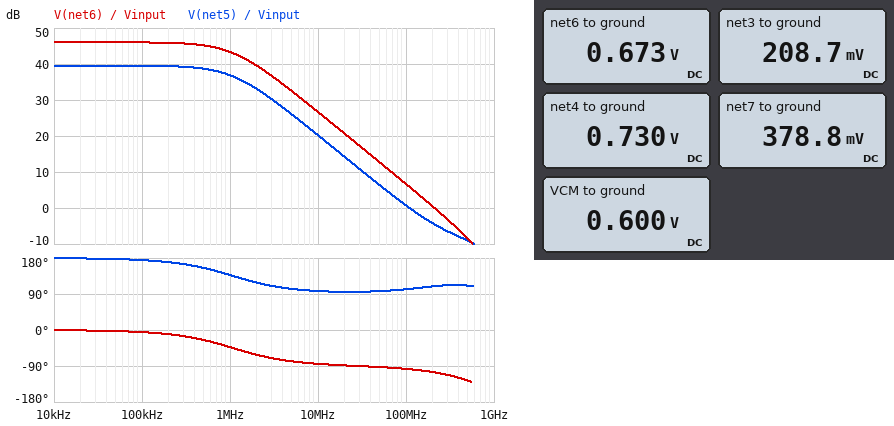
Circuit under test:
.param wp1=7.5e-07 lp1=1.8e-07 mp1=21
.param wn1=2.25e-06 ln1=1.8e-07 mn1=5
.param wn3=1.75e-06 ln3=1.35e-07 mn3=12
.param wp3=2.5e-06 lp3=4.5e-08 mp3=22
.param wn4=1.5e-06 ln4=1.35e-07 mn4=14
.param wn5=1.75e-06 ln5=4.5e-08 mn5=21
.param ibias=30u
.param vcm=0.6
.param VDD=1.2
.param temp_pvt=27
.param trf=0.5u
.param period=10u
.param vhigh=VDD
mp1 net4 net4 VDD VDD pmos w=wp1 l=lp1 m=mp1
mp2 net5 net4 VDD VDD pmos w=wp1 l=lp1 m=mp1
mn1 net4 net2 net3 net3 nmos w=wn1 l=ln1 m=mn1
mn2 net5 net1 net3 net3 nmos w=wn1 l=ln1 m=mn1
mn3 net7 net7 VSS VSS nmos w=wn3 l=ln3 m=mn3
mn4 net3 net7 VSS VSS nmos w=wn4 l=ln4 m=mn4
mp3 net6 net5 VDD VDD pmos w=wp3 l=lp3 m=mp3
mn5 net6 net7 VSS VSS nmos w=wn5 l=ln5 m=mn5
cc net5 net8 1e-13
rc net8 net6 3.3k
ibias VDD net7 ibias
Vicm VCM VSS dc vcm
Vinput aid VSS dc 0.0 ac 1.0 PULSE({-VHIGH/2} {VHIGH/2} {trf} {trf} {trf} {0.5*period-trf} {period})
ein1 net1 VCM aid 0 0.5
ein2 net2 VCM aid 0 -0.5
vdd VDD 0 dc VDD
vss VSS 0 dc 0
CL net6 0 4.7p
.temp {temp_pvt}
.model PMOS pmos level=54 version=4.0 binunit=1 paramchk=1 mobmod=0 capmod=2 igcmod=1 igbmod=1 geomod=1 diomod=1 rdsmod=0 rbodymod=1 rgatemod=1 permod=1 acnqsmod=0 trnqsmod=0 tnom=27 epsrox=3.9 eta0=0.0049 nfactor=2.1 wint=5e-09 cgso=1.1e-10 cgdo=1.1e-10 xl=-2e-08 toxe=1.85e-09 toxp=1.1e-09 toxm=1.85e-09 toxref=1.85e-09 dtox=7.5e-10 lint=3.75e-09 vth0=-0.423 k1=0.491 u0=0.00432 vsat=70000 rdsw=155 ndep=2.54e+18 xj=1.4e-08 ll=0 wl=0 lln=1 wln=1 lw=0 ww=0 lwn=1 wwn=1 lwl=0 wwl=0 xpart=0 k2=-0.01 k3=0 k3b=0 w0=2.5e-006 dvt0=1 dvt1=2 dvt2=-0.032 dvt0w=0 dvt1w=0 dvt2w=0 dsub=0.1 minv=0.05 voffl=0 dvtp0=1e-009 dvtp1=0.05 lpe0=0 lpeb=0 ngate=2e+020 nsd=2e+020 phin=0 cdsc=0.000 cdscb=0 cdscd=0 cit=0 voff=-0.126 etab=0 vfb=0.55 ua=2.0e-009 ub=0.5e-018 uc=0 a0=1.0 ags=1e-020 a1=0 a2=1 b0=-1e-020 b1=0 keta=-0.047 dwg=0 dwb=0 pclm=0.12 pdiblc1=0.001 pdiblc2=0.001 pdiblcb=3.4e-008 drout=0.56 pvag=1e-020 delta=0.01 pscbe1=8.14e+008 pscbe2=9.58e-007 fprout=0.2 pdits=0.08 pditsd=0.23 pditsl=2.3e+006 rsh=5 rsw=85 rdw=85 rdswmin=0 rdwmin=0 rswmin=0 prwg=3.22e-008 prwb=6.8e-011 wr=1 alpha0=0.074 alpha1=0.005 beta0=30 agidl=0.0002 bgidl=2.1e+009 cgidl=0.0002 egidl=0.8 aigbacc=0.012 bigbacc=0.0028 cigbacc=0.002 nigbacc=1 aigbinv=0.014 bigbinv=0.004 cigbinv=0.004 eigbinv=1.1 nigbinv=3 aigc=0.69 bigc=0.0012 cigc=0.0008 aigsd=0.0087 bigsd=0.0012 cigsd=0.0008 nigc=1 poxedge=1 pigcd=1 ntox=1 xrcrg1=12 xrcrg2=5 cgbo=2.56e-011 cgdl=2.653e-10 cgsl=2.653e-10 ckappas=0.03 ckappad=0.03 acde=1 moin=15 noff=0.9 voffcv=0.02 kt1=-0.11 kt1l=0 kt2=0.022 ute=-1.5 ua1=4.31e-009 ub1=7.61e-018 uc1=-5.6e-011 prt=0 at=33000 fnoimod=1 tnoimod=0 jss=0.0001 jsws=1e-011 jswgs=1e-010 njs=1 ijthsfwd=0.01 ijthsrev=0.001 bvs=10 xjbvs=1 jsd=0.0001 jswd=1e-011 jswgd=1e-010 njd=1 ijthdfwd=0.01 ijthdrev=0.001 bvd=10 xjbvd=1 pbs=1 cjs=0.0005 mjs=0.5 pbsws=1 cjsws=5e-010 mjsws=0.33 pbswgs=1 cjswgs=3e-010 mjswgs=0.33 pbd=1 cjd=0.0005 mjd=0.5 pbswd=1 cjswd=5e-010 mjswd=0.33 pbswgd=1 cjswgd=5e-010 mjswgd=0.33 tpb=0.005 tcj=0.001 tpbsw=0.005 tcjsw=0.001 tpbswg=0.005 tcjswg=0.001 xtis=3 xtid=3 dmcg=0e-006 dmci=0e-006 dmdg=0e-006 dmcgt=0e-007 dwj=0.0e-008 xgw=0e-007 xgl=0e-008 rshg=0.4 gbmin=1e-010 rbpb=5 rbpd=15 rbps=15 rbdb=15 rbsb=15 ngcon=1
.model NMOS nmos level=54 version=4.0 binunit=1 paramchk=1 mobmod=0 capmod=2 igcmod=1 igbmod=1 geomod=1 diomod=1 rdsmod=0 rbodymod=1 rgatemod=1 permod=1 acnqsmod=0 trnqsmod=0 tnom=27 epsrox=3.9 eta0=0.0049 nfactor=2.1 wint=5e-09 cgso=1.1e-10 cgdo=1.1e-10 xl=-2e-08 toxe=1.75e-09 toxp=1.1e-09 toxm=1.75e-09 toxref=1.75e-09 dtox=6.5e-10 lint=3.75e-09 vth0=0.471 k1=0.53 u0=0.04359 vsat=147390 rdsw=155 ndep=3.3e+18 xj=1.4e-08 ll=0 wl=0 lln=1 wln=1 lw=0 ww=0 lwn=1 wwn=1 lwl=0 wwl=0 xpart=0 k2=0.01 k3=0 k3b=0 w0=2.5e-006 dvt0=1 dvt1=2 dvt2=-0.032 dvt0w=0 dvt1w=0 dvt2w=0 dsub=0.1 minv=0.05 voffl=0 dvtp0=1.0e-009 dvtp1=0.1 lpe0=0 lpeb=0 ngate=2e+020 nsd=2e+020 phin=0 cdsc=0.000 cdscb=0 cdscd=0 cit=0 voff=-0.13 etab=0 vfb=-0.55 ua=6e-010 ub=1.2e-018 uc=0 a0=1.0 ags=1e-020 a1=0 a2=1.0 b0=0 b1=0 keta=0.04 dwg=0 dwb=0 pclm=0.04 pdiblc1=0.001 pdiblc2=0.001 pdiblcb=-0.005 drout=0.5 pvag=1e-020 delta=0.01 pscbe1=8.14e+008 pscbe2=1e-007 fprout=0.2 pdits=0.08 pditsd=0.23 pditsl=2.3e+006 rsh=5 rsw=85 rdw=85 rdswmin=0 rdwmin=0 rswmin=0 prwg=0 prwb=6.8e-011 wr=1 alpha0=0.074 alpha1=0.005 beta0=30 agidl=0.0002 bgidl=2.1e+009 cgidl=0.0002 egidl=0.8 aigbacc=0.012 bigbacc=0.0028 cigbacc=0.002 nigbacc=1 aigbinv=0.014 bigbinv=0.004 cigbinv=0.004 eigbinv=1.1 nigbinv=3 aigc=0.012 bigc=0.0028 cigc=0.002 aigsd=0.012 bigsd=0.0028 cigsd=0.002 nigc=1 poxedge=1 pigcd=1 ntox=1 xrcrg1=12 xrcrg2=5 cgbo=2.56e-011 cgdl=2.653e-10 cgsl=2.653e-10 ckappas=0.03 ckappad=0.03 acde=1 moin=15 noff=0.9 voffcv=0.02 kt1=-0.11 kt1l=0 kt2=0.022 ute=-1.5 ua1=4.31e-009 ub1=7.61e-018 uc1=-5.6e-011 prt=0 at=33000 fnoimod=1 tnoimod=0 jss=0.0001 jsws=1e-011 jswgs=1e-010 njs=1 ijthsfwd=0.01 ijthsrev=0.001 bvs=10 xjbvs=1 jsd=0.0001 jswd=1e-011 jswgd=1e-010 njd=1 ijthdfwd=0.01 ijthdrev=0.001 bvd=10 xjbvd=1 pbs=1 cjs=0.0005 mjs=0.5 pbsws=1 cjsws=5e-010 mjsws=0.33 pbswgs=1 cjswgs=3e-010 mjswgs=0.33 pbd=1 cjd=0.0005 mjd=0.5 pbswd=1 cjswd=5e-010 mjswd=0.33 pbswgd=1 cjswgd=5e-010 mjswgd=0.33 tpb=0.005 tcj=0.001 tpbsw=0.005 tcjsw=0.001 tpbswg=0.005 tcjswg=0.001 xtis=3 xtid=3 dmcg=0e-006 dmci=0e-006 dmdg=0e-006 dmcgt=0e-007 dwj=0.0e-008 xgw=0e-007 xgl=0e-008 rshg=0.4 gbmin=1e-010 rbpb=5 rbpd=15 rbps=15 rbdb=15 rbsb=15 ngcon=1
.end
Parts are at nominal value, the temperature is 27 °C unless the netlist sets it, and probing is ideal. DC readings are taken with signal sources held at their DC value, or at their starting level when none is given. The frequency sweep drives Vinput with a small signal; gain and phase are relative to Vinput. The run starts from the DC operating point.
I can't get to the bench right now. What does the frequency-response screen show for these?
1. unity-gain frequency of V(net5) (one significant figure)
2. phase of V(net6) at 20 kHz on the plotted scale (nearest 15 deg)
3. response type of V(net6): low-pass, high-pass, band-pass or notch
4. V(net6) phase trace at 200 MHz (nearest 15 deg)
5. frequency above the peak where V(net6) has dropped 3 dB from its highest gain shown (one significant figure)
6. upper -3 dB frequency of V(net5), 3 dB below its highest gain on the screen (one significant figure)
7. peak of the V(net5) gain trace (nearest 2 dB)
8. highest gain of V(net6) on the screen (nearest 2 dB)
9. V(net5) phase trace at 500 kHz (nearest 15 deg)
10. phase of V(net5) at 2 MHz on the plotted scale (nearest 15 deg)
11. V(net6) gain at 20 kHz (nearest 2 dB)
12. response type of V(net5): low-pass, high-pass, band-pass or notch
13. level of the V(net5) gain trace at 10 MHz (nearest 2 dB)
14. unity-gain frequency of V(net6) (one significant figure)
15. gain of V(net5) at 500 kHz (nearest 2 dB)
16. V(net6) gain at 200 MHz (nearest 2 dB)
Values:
100 MHz
0 deg
low-pass
-105 deg
1 MHz
1 MHz
40 dB
46 dB
150 deg
120 deg
46 dB
low-pass
20 dB
200 MHz
38 dB
0 dB
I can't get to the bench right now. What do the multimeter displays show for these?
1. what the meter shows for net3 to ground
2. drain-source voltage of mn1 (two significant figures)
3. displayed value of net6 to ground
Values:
208.7 mV
520 mV
0.673 V
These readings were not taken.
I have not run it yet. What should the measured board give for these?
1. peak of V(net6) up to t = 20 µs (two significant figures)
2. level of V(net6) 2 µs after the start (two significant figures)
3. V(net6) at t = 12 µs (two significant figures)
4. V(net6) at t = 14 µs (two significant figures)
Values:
1.1 V
1.1 V
1.1 V
1.1 V
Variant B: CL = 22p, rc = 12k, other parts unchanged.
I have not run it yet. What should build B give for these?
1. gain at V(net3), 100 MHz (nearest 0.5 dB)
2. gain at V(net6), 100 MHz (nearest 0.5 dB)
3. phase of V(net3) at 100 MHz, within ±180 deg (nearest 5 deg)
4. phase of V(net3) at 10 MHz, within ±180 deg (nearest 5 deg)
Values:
-29.5 dB
7.0 dB
160 deg
145 deg
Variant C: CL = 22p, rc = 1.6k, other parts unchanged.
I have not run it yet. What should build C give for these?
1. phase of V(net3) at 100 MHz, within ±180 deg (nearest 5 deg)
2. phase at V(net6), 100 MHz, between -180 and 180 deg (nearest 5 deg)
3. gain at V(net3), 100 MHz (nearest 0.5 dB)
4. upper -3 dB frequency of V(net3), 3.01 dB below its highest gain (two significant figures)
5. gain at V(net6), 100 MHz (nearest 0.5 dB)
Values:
140 deg
-125 deg
-31.5 dB
1.1 MHz
5.0 dB
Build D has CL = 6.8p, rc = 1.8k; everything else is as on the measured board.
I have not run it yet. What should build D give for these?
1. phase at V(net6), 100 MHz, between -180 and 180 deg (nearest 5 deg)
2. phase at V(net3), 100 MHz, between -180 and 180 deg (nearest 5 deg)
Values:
-105 deg
150 deg
